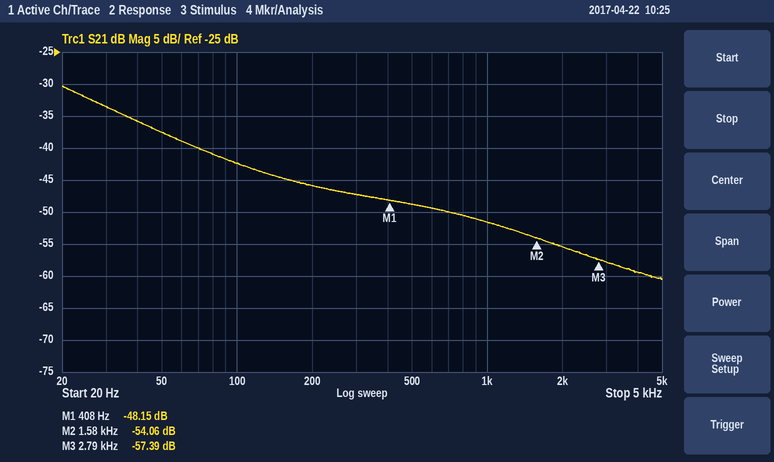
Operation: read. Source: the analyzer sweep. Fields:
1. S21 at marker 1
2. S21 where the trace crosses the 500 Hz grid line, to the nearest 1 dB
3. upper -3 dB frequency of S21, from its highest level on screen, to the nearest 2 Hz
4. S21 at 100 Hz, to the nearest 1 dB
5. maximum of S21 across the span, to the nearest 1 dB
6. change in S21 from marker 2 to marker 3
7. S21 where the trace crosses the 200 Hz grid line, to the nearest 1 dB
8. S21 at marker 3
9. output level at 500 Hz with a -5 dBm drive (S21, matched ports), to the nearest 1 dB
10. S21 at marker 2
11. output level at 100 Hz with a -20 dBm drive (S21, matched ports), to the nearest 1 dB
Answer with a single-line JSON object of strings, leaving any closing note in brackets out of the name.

{"S21 at marker 1": "-48.15 dB", "S21 where the trace crosses the 500 Hz grid line, to the nearest 1 dB": "-49 dB", "upper -3 dB frequency of S21, from its highest level on screen, to the nearest 2 Hz": "30 Hz", "S21 at 100 Hz, to the nearest 1 dB": "-42 dB", "maximum of S21 across the span, to the nearest 1 dB": "-30 dB", "change in S21 from marker 2 to marker 3": "-3.33 dB", "S21 where the trace crosses the 200 Hz grid line, to the nearest 1 dB": "-46 dB", "S21 at marker 3": "-57.39 dB", "output level at 500 Hz with a -5 dBm drive (S21, matched ports), to the nearest 1 dB": "-54 dBm", "S21 at marker 2": "-54.06 dB", "output level at 100 Hz with a -20 dBm drive (S21, matched ports), to the nearest 1 dB": "-62 dBm"}
